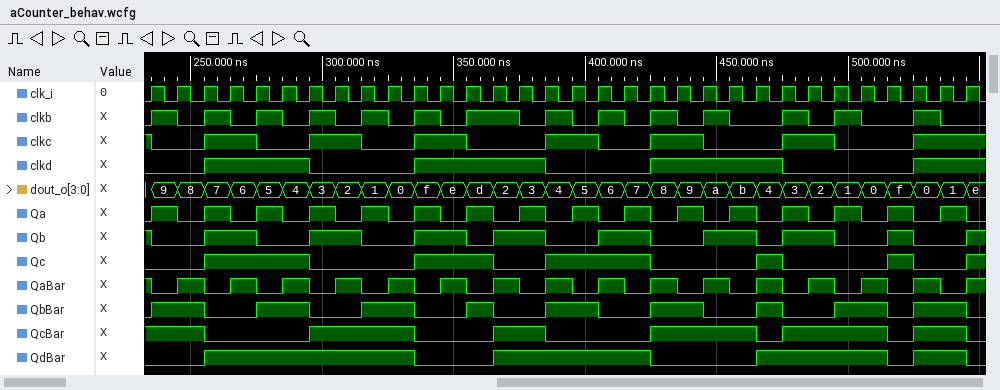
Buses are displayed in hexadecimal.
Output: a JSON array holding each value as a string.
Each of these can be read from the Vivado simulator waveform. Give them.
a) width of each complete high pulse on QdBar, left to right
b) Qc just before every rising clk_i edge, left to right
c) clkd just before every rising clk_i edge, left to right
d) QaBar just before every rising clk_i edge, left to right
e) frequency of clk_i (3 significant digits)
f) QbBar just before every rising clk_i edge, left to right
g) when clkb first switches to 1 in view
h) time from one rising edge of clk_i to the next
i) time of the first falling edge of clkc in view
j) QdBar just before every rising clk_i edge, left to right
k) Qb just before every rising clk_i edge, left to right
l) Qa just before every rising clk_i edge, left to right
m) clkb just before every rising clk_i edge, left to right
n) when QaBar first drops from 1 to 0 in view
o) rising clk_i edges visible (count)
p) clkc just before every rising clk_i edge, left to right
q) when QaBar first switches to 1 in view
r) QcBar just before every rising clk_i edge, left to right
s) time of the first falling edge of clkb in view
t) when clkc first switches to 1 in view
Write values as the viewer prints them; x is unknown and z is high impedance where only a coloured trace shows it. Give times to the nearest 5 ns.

["80 ns, 60 ns, 50 ns, 20 ns", "0 0 0 1 1 1 1 0 0 0 0 1 1 1 0 0 1 1 1 1 0 0 0 0 1 0 0 0 0 1 0 0", "0 0 0 1 1 1 1 0 0 0 0 1 1 1 1 1 0 0 0 0 1 1 1 1 1 0 0 0 0 0 1 1", "1 0 1 0 1 0 1 0 1 0 1 0 1 0 1 0 1 0 1 0 1 0 1 0 1 0 1 0 1 0 1 0", "100 MHz", "0 1 1 0 0 1 1 0 0 1 1 0 0 1 0 0 1 1 0 0 1 1 0 0 1 0 0 1 1 0 1 1", "235 ns", "10 ns", "235 ns", "0 0 0 1 1 1 1 1 1 1 1 0 0 0 1 1 1 1 1 1 0 0 0 0 1 1 1 1 1 0 1 1", "1 0 0 1 1 0 0 1 1 0 0 1 1 0 1 1 0 0 1 1 0 0 1 1 0 1 1 0 0 1 0 0", "0 1 0 1 0 1 0 1 0 1 0 1 0 1 0 1 0 1 0 1 0 1 0 1 0 1 0 1 0 1 0 1", "0 1 0 1 0 1 0 1 0 1 0 1 0 1 1 0 1 0 1 0 1 0 1 0 0 1 0 1 0 0 1 0", "235 ns", "32", "1 0 0 1 1 0 0 1 1 0 0 1 1 0 0 0 1 1 0 0 1 1 0 0 0 1 1 0 0 0 1 1", "245 ns", "1 1 1 0 0 0 0 1 1 1 1 0 0 0 1 1 0 0 0 0 1 1 1 1 0 1 1 1 1 0 1 1", "245 ns", "255 ns"]
